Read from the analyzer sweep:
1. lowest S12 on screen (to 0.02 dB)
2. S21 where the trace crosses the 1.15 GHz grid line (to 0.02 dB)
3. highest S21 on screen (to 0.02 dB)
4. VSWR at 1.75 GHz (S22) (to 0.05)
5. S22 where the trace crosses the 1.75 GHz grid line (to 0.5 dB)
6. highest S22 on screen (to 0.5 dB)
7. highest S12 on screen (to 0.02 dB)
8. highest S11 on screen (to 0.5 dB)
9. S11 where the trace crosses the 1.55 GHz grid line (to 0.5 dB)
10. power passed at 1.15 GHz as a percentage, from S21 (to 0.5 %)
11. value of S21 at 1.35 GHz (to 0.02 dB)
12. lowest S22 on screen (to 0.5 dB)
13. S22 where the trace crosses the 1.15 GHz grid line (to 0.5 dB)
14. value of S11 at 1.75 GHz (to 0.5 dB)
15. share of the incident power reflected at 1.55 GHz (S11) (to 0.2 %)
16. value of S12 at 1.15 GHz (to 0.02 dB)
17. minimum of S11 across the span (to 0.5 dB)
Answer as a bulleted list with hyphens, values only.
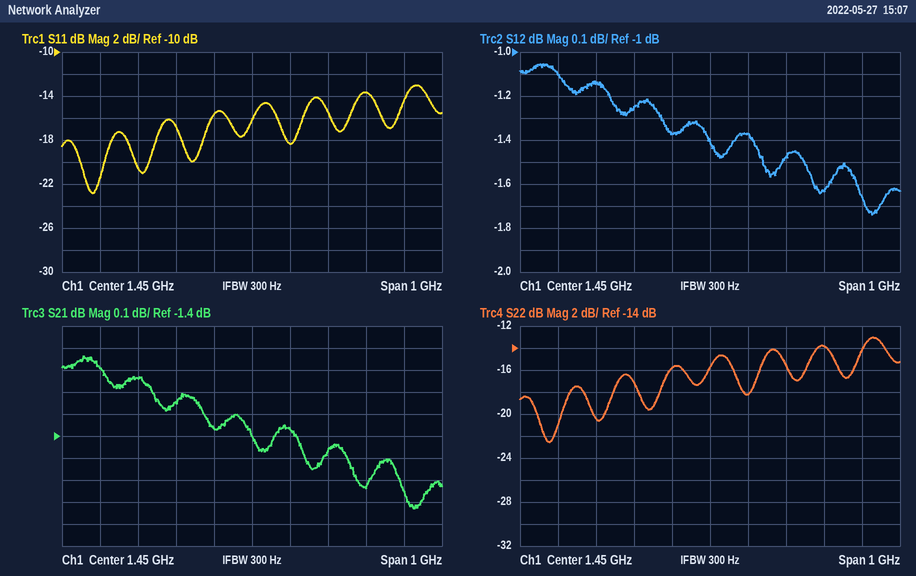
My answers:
- -1.74 dB
- -1.14 dB
- -1.04 dB
- 1.50
- -14.0 dB
- -13.0 dB
- -1.06 dB
- -13.0 dB
- -18.5 dB
- 77.0 %
- -1.36 dB
- -22.5 dB
- -20.5 dB
- -13.5 dB
- 1.4 %
- -1.14 dB
- -23.0 dB
